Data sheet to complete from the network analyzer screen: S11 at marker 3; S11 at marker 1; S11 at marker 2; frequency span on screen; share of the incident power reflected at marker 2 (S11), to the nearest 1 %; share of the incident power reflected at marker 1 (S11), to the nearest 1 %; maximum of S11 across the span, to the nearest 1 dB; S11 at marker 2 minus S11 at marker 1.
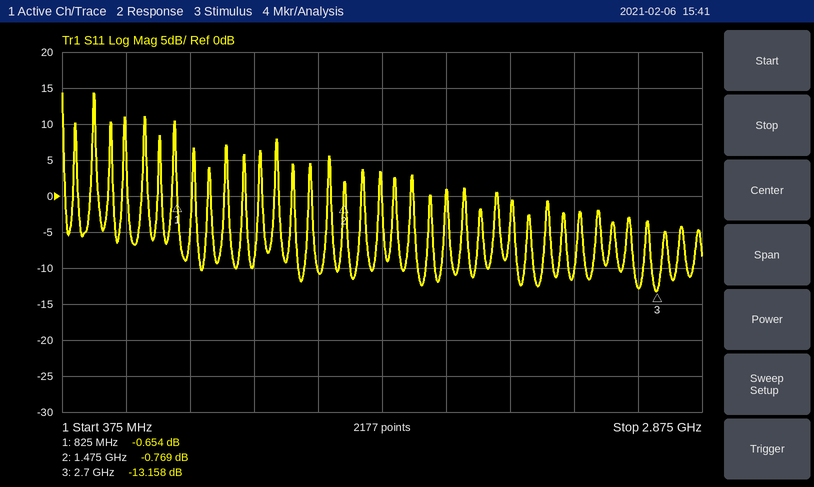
-13.158 dB
-0.654 dB
-0.769 dB
2.5 GHz
84 %
86 %
14 dB
-0.115 dB
